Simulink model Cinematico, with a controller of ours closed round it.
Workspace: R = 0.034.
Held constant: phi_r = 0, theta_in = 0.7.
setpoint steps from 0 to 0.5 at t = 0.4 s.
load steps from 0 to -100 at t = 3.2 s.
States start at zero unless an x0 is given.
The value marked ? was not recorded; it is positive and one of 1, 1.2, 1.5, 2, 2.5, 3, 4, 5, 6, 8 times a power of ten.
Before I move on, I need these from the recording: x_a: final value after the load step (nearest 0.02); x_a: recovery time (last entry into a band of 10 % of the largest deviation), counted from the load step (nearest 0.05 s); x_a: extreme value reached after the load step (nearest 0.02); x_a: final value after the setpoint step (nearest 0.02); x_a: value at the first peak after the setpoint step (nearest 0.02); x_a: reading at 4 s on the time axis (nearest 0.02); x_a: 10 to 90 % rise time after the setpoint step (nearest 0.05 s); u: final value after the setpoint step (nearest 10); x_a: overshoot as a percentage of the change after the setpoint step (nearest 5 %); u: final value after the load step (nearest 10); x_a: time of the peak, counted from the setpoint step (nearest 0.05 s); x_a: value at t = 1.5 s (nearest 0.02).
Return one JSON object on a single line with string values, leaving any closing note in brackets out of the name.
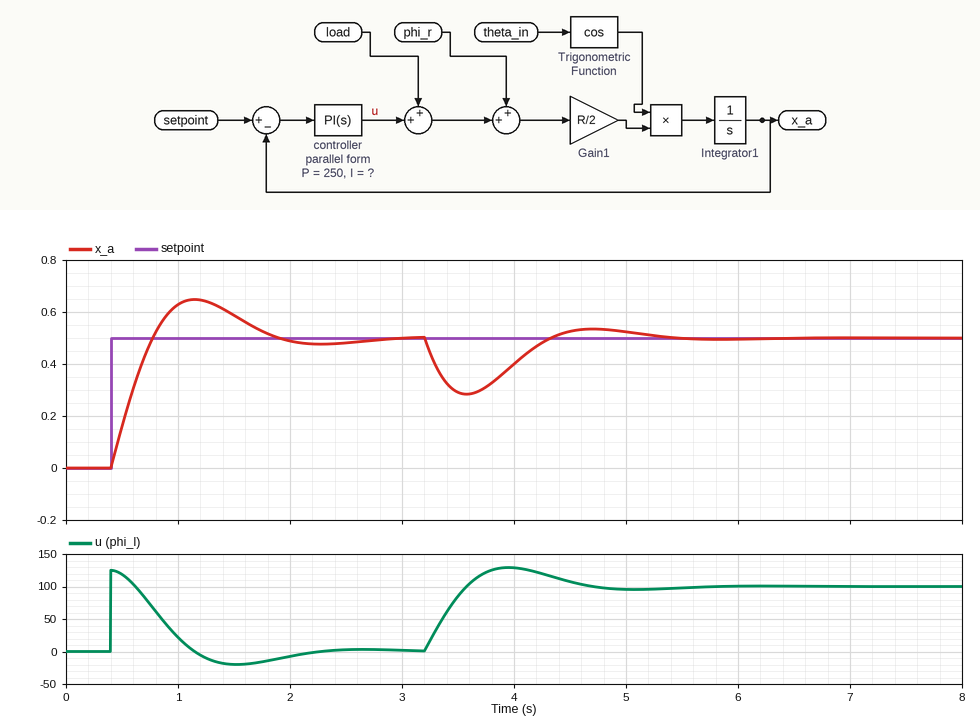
{"x_a: final value after the load step": "0.50", "x_a: recovery time (last entry into a band of 10 % of the largest deviation), counted from the load step": "1.85 s", "x_a: extreme value reached after the load step": "0.28", "x_a: final value after the setpoint step": "0.50", "x_a: value at the first peak after the setpoint step": "0.64", "x_a: reading at 4 s on the time axis": "0.40", "x_a: 10 to 90 % rise time after the setpoint step": "0.30 s", "u: final value after the setpoint step": "0", "x_a: overshoot as a percentage of the change after the setpoint step": "30 %", "u: final value after the load step": "100", "x_a: time of the peak, counted from the setpoint step": "0.75 s", "x_a: value at t = 1.5 s": "0.58"}
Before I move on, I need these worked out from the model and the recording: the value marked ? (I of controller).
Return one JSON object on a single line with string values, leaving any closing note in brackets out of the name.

{"the value marked ?": "800"}
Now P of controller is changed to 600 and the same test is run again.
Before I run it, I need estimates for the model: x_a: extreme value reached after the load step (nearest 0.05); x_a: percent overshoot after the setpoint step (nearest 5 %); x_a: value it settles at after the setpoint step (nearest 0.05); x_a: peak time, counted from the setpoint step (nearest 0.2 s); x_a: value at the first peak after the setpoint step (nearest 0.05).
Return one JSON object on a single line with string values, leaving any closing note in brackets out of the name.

{"x_a: extreme value reached after the load step": "0.35", "x_a: percent overshoot after the setpoint step": "10 %", "x_a: value it settles at after the setpoint step": "0.50", "x_a: peak time, counted from the setpoint step": "0.6 s", "x_a: value at the first peak after the setpoint step": "0.55"}
